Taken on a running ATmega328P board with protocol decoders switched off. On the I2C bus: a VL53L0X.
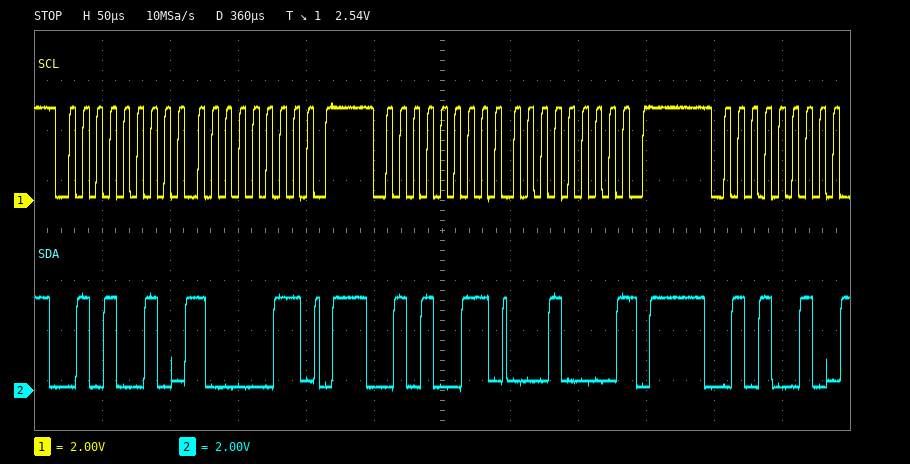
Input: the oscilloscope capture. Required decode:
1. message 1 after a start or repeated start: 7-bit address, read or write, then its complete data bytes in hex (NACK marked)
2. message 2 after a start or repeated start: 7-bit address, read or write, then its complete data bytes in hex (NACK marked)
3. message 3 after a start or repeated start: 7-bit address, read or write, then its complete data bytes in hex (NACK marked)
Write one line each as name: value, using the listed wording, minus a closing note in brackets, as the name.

message 1 after a start or repeated start: 7-bit address, read or write, then its complete data bytes in hex: 0x29 write: 83
message 2 after a start or repeated start: 7-bit address, read or write, then its complete data bytes in hex: 0x29 read: 10 NACK
message 3 after a start or repeated start: 7-bit address, read or write, then its complete data bytes in hex: 0x29 write
